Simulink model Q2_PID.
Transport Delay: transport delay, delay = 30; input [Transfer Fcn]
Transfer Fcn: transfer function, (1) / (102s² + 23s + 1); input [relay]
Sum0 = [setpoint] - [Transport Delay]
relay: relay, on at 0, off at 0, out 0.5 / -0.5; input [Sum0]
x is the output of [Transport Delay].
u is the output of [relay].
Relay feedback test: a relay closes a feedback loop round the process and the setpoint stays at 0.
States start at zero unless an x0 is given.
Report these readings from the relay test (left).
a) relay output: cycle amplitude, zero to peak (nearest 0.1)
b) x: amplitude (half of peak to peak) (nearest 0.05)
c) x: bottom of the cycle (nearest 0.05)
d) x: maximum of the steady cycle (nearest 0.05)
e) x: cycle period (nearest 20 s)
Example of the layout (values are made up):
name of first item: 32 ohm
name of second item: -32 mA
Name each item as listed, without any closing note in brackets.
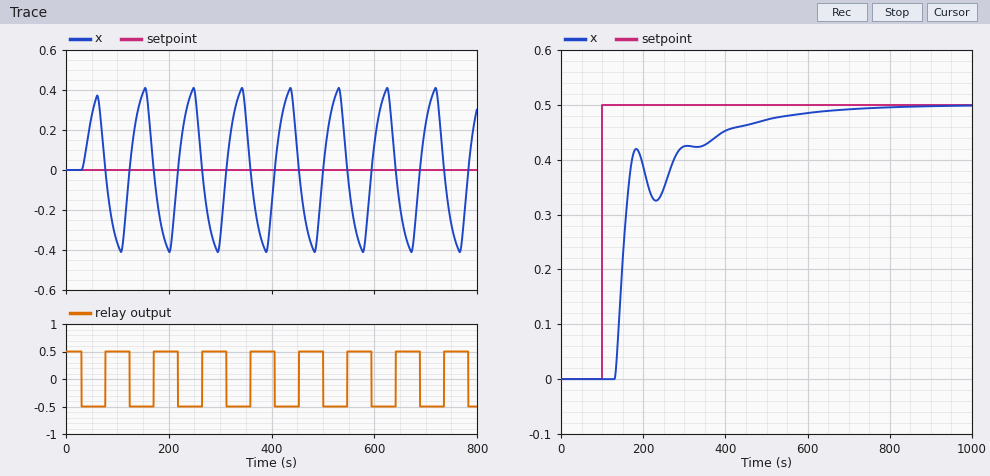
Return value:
relay output: cycle amplitude, zero to peak: 0.5
x: amplitude (half of peak to peak): 0.40
x: bottom of the cycle: -0.40
x: maximum of the steady cycle: 0.40
x: cycle period: 100 s
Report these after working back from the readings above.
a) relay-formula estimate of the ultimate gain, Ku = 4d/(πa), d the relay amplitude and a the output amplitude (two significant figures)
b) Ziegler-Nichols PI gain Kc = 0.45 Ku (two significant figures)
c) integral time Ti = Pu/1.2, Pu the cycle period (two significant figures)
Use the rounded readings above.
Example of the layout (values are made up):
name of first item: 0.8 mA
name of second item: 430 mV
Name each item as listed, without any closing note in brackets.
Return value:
relay-formula estimate of the ultimate gain, Ku = 4d/(πa), d the relay amplitude and a the output amplitude: 1.6
Ziegler-Nichols PI gain Kc = 0.45 Ku: 0.72
integral time Ti = Pu/1.2, Pu the cycle period: 83 s
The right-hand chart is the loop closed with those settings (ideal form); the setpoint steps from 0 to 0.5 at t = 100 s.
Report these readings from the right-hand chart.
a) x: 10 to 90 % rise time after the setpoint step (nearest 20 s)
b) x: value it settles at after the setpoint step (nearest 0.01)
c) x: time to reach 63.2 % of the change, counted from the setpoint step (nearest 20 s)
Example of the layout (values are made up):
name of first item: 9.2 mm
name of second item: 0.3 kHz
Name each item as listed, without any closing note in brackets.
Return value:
x: 10 to 90 % rise time after the setpoint step: 260 s
x: value it settles at after the setpoint step: 0.50
x: time to reach 63.2 % of the change, counted from the setpoint step: 60 s
